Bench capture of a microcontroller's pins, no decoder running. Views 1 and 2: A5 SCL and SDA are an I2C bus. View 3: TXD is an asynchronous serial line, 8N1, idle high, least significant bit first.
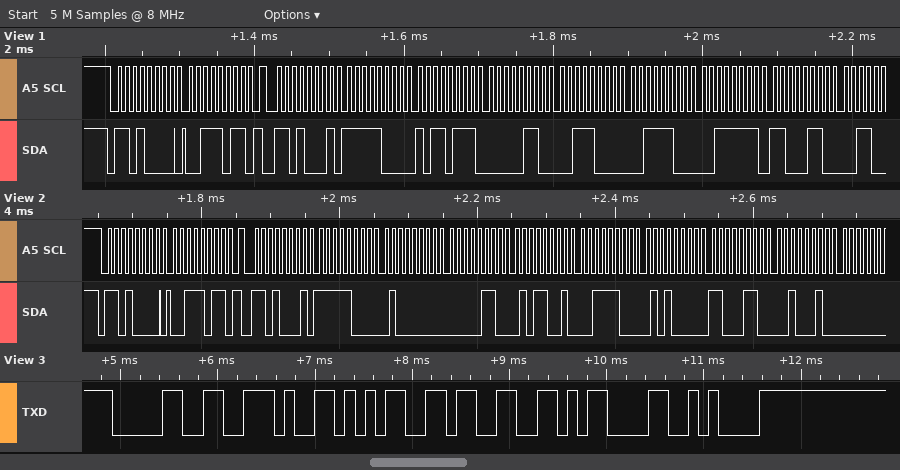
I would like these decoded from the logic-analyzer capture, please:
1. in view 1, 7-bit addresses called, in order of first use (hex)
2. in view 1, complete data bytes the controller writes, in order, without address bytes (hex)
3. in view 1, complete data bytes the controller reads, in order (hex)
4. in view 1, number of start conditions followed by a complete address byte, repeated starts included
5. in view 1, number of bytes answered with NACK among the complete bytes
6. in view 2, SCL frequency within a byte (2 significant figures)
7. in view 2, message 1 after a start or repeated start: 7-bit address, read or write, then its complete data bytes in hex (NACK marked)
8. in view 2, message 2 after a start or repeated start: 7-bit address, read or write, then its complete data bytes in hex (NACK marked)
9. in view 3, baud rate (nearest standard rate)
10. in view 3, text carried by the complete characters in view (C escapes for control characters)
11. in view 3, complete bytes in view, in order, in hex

0x68
3B
F8 B7 06 38 3C 3F C6
2
0
100 kHz
0x68 write: 3B
0x68 read: F8 40 06 59 3C 50 C6 22
9600 baud
"0.53\r\n"
30 2E 35 33 0D 0A
